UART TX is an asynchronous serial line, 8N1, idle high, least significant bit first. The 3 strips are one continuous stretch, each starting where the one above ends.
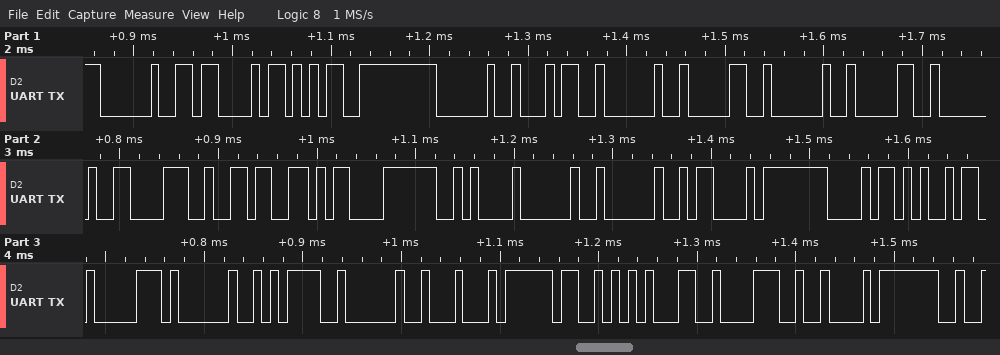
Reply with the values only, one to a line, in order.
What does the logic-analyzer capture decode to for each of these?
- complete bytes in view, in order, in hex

0x20 0x43 0x35 0x20 0x34 0x20 0x30 0x20 0x30 0x20 0x38 0x36 0x0D 0x0A 0x20 0x20 0x43 0x68 0x69 0x70 0x20 0x3D 0x20 0x44 0x53 0x31 0x38 0x42
